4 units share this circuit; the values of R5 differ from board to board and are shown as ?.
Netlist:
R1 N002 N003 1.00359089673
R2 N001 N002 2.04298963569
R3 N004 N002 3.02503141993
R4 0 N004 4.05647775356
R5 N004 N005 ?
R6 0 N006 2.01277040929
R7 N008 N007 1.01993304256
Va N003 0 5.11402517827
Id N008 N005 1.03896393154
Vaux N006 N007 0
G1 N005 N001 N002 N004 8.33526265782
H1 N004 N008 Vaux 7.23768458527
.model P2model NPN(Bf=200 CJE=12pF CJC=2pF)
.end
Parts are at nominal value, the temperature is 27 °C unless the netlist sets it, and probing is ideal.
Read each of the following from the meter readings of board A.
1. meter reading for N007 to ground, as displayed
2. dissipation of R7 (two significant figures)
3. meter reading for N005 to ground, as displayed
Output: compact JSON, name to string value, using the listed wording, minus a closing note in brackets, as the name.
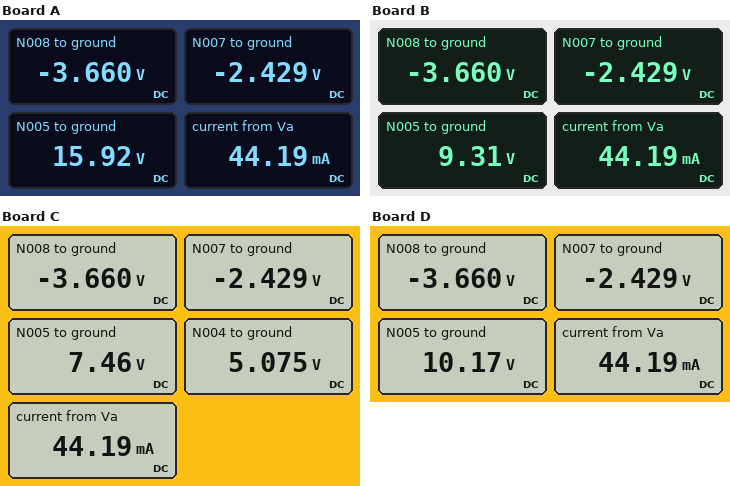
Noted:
{"meter reading for N007 to ground, as displayed": "-2.429 V", "dissipation of R7": "1.5 W", "meter reading for N005 to ground, as displayed": "15.92 V"}
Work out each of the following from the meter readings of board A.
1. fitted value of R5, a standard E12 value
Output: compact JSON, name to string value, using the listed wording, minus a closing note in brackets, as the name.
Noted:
{"fitted value of R5, a standard E12 value": "10 Ω"}
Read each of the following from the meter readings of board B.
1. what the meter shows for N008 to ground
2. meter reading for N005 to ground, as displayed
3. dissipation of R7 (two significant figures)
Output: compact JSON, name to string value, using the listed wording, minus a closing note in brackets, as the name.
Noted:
{"what the meter shows for N008 to ground": "-3.660 V", "meter reading for N005 to ground, as displayed": "9.31 V", "dissipation of R7": "1.5 W"}
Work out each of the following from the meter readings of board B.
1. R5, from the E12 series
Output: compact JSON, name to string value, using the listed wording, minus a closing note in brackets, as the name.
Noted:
{"R5, from the E12 series": "3.9 Ω"}
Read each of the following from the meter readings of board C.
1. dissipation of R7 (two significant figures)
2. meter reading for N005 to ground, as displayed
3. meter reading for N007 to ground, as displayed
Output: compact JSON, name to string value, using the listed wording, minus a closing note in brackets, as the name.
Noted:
{"dissipation of R7": "1.5 W", "meter reading for N005 to ground, as displayed": "7.46 V", "meter reading for N007 to ground, as displayed": "-2.429 V"}
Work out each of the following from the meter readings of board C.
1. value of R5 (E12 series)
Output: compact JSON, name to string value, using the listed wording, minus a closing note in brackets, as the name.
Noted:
{"value of R5": "2.2 Ω"}
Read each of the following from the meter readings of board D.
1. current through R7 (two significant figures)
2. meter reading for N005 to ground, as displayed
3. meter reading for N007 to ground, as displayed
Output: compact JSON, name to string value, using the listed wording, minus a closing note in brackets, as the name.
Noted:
{"current through R7": "1.2 A", "meter reading for N005 to ground, as displayed": "10.17 V", "meter reading for N007 to ground, as displayed": "-2.429 V"}
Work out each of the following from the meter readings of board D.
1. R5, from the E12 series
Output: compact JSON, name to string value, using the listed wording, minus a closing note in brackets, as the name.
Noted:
{"R5, from the E12 series": "4.7 Ω"}
